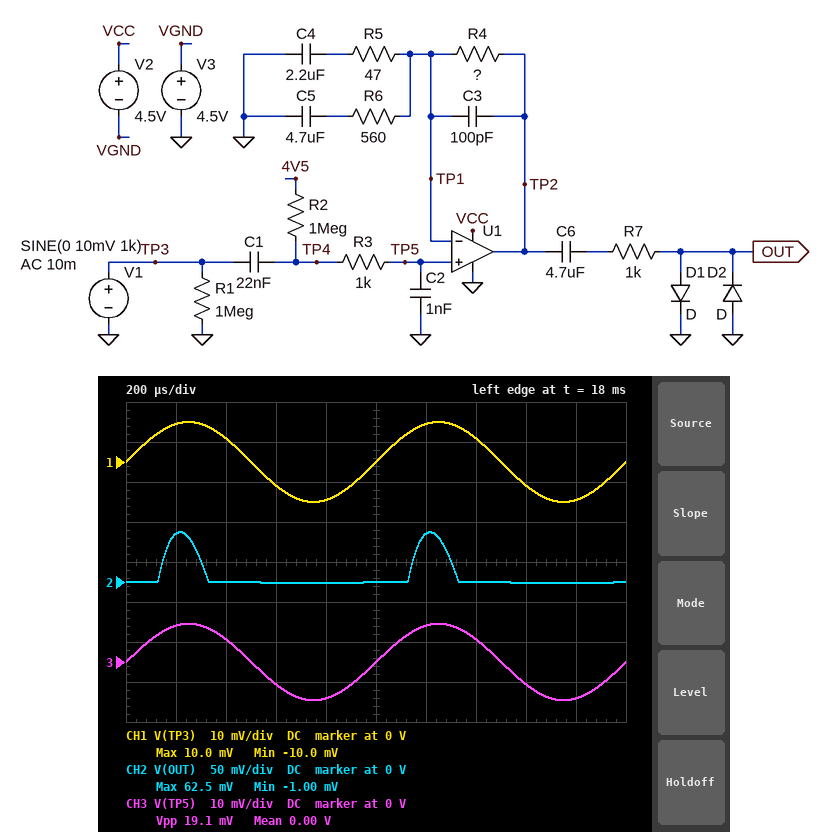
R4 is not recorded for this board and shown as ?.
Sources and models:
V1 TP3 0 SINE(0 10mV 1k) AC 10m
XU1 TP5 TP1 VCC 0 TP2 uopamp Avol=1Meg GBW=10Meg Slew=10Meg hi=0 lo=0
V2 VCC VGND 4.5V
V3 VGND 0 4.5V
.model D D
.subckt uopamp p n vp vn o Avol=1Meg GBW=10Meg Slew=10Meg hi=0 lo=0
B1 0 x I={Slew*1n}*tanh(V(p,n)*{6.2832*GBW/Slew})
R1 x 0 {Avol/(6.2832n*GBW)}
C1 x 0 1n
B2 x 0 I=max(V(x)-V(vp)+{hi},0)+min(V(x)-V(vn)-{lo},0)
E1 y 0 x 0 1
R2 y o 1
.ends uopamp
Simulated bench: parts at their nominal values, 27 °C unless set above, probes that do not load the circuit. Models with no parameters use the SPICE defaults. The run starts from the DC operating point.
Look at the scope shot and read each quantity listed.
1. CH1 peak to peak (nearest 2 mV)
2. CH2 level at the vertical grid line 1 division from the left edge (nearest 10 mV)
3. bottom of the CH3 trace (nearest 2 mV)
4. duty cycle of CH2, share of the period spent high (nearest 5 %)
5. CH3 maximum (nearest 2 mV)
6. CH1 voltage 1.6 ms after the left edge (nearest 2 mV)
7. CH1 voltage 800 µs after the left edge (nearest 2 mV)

20 mV
60 mV
-10 mV
15 %
10 mV
-6 mV
-10 mV
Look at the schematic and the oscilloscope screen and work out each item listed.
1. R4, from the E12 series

1.5 kΩ
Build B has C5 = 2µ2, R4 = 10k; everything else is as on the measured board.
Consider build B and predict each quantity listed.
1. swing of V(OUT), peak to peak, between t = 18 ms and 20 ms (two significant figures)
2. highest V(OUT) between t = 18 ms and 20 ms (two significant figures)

130 mV
120 mV
